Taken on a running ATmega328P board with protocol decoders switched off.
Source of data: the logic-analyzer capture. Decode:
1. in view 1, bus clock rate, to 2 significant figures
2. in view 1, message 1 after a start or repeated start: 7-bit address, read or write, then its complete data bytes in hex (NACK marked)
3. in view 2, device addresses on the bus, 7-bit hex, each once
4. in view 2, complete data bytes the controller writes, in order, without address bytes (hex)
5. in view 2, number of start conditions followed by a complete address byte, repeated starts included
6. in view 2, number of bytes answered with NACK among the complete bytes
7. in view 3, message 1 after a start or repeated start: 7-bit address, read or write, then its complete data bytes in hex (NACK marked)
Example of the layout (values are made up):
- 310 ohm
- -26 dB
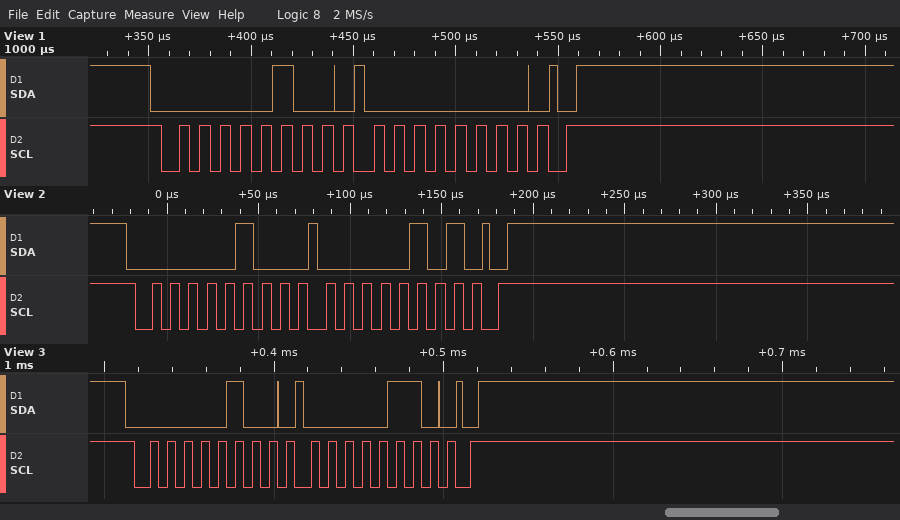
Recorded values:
- 100 kHz
- 0x02 write: 00
- 0x02
- 05
- 1
- 0
- 0x02 write: 06
